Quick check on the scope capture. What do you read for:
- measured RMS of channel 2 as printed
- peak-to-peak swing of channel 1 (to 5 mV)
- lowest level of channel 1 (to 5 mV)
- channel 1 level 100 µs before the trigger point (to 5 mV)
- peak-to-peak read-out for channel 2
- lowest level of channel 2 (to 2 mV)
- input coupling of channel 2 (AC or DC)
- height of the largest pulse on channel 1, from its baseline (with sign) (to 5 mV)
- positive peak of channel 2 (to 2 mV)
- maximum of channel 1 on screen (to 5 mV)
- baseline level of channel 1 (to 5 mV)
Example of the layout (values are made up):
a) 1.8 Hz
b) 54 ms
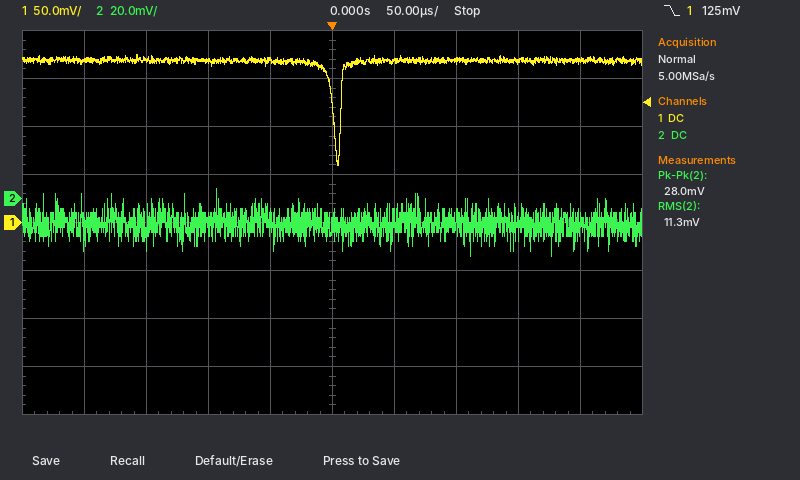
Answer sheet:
a) 11.3 mV
b) 115 mV
c) 60 mV
d) 170 mV
e) 28.0 mV
f) -24 mV
g) DC
h) -110 mV
i) 4 mV
j) 175 mV
k) 170 mV
